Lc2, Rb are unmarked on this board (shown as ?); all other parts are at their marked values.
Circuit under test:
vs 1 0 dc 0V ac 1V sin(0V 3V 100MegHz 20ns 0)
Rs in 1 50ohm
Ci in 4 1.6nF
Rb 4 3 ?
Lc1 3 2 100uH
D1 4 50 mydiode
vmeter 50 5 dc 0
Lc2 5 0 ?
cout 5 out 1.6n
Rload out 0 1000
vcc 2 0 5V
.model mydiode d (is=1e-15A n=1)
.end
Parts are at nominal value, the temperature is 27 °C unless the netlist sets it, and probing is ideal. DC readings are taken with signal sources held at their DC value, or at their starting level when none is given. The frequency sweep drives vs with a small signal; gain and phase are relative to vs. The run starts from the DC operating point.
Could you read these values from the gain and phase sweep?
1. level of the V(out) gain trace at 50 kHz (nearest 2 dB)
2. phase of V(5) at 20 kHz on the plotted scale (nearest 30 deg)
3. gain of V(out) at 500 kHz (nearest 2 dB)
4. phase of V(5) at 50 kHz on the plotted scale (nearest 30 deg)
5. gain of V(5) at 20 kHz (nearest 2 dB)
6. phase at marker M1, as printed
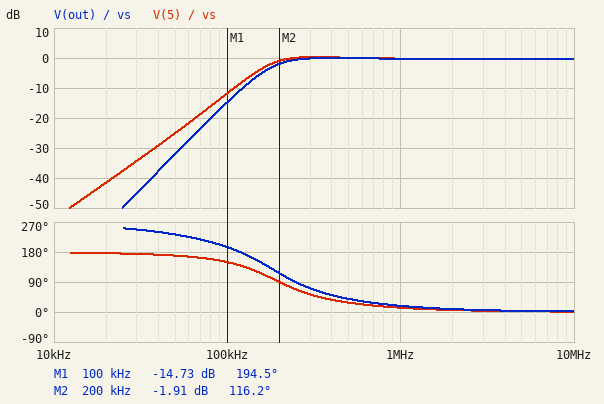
-32 dB
180 deg
0 dB
180 deg
-42 dB
194.5 deg
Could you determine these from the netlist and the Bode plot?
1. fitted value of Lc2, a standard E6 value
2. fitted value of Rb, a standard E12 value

330 µH
820 Ω
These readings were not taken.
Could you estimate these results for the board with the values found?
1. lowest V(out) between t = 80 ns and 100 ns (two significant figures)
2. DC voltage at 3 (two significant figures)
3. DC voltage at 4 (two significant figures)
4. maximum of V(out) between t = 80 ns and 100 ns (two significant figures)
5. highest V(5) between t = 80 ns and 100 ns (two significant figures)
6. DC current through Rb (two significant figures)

-2.8 V
5.0 V
1.5 V
2.8 V
2.8 V
4.2 mA
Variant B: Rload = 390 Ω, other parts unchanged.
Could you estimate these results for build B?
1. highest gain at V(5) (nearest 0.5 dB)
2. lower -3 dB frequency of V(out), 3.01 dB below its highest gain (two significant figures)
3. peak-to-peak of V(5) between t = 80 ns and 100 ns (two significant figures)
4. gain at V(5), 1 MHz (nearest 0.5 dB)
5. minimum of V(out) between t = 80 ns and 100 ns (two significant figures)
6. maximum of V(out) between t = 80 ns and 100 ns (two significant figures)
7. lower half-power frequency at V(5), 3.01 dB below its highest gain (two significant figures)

-1.0 dB
350 kHz
4.3 V
-1.5 dB
-1.7 V
2.6 V
140 kHz
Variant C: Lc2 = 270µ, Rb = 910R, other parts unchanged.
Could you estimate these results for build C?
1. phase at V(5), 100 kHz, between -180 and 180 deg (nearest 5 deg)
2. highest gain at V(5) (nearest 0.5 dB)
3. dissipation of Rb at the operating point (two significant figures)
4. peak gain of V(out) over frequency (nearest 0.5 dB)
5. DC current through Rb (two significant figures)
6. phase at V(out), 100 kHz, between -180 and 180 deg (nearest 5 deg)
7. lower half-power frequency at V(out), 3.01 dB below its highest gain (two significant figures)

155 deg
1.0 dB
13 mW
0.5 dB
3.8 mA
-160 deg
190 kHz
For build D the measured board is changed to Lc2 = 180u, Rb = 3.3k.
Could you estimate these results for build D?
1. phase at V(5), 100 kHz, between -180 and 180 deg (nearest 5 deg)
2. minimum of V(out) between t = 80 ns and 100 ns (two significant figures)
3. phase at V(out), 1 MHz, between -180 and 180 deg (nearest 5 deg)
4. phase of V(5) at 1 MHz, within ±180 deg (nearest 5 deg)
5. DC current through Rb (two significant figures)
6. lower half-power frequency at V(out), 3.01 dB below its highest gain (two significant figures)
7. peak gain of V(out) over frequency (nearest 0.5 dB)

170 deg
-1.3 V
15 deg
10 deg
1.1 mA
230 kHz
3.5 dB
